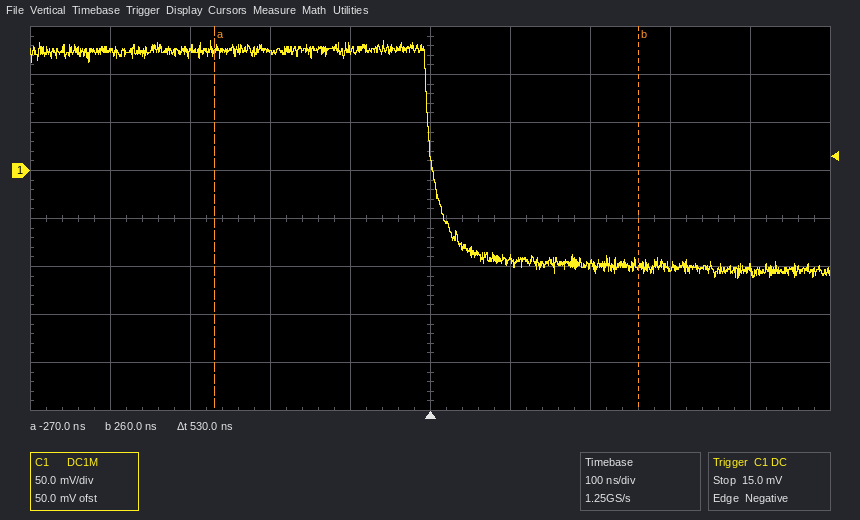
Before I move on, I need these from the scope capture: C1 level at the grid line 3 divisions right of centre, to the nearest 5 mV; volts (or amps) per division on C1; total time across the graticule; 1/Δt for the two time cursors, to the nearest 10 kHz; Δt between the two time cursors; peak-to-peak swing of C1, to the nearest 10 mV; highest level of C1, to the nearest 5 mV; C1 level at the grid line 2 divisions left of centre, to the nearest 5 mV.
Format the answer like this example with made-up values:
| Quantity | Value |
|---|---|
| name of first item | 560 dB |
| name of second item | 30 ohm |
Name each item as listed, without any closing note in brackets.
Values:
| Quantity | Value |
|---|---|
| C1 level at the grid line 3 divisions right of centre, to the nearest 5 mV | -100 mV |
| volts (or amps) per division on C1 | 50 mV |
| total time across the graticule | 1 µs |
| 1/Δt for the two time cursors, to the nearest 10 kHz | 1.89 MHz |
| Δt between the two time cursors | 530 ns |
| peak-to-peak swing of C1, to the nearest 10 mV | 250 mV |
| highest level of C1, to the nearest 5 mV | 135 mV |
| C1 level at the grid line 2 divisions left of centre, to the nearest 5 mV | 125 mV |
